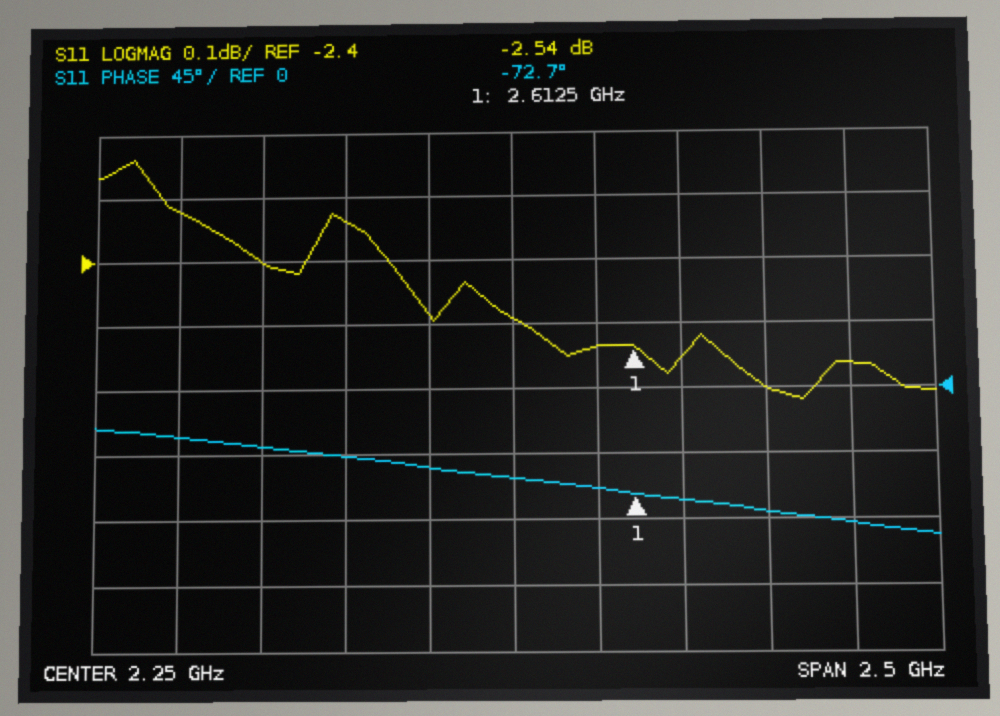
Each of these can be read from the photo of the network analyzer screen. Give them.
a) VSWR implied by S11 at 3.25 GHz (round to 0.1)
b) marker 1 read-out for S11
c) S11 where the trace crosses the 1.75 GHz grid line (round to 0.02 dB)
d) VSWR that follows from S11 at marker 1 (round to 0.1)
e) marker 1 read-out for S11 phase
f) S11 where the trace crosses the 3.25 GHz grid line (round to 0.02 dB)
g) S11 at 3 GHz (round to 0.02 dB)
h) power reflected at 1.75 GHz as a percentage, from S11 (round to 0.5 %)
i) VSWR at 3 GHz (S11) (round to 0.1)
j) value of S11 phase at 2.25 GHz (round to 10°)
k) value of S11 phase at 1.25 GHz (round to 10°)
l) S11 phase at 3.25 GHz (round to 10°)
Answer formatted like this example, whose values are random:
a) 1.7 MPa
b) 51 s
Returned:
a) 6.8
b) -2.54 dB
c) -2.34 dB
d) 6.9
e) -72.7°
f) -2.56 dB
g) -2.60 dB
h) 58.5 %
i) 6.7
j) -60°
k) -30°
l) -90°
